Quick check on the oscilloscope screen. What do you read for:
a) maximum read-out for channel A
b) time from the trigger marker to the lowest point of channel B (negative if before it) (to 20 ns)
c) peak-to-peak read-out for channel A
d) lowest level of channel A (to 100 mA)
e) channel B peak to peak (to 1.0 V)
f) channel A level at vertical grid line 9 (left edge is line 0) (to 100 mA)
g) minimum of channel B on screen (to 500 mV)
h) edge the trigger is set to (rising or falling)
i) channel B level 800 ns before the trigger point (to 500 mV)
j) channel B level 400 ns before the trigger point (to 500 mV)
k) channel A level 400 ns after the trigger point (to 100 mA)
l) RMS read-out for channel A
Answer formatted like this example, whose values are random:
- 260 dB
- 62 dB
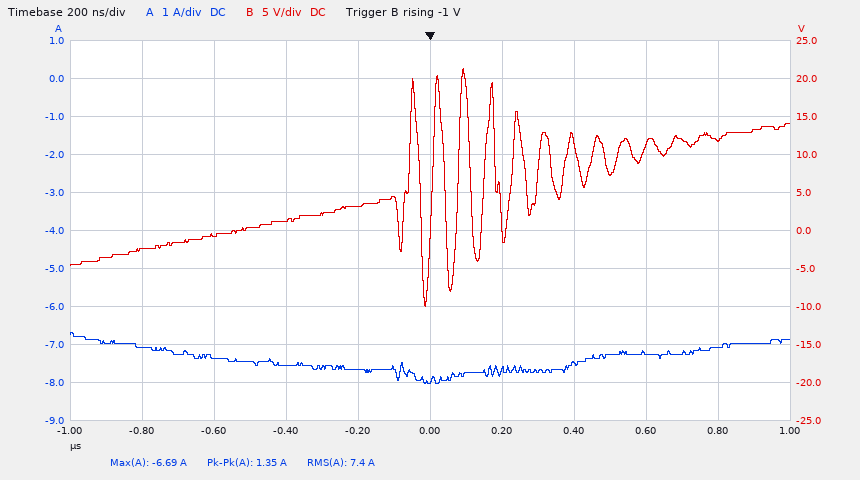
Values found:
- -6.69 A
- -20 ns
- 1.35 A
- -8.0 A
- 31.0 V
- -7.1 A
- -10.0 V
- rising
- -2.5 V
- 1.5 V
- -7.5 A
- 7.4 A
